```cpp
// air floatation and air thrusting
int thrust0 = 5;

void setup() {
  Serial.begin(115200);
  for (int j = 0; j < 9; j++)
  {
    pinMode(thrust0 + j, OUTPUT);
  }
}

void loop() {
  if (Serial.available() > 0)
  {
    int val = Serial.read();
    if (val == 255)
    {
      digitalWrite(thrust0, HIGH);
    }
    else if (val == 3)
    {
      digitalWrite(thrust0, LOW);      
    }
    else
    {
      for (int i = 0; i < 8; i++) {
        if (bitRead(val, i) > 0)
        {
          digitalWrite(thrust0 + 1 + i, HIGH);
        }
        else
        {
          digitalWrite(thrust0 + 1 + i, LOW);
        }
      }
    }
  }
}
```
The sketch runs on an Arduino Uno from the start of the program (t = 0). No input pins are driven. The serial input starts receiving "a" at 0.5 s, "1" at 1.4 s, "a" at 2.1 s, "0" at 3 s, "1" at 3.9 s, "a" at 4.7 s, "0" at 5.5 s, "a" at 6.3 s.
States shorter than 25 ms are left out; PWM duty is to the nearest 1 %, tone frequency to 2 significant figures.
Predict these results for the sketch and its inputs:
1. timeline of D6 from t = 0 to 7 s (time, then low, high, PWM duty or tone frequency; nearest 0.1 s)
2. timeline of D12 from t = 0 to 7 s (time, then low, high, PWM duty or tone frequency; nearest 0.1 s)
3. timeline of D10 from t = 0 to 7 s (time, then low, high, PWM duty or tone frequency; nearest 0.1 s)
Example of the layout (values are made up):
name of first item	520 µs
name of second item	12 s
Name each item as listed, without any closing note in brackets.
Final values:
timeline of D6 from t = 0 to 7 s	0 s low; 0.5 s high; 3 s low; 3.9 s high; 5.5 s low; 6.3 s high
timeline of D12 from t = 0 to 7 s	0 s low; 0.5 s high; 1.4 s low; 2.1 s high; 3 s low; 4.7 s high; 5.5 s low; 6.3 s high
timeline of D10 from t = 0 to 7 s	0 s low; 1.4 s high; 2.1 s low; 3 s high; 4.7 s low; 5.5 s high; 6.3 s low
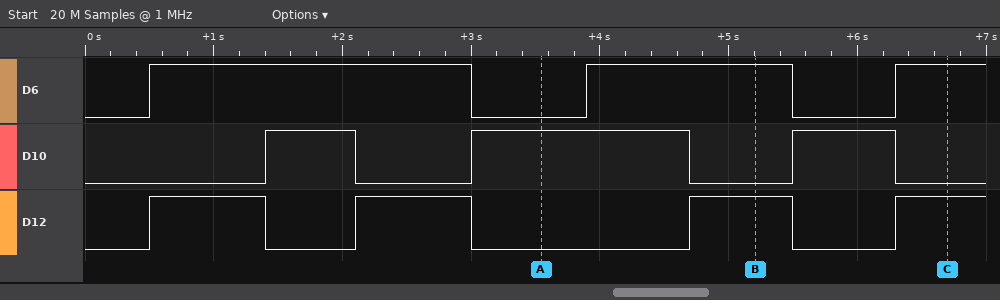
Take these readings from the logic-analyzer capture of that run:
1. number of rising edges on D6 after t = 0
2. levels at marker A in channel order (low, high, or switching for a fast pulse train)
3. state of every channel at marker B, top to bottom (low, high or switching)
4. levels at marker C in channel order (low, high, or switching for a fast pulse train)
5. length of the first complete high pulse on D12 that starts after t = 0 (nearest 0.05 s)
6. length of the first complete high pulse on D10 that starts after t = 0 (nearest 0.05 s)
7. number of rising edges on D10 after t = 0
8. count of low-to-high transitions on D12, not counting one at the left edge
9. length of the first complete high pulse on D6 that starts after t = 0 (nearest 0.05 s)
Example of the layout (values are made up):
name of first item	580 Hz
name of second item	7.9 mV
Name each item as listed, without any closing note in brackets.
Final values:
number of rising edges on D6 after t = 0	3
levels at marker A in channel order	D6 low, D10 high, D12 low
state of every channel at marker B, top to bottom	D6 high, D10 low, D12 high
levels at marker C in channel order	D6 high, D10 low, D12 high
length of the first complete high pulse on D12 that starts after t = 0	0.90 s
length of the first complete high pulse on D10 that starts after t = 0	0.70 s
number of rising edges on D10 after t = 0	3
count of low-to-high transitions on D12, not counting one at the left edge	4
length of the first complete high pulse on D6 that starts after t = 0	2.50 s
